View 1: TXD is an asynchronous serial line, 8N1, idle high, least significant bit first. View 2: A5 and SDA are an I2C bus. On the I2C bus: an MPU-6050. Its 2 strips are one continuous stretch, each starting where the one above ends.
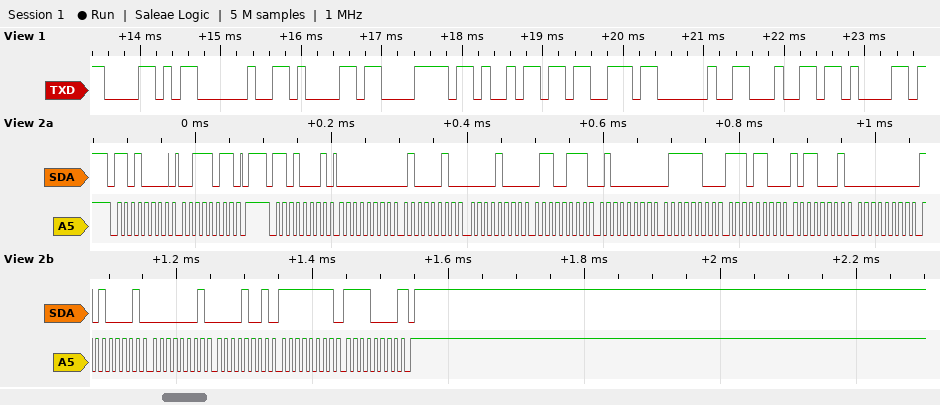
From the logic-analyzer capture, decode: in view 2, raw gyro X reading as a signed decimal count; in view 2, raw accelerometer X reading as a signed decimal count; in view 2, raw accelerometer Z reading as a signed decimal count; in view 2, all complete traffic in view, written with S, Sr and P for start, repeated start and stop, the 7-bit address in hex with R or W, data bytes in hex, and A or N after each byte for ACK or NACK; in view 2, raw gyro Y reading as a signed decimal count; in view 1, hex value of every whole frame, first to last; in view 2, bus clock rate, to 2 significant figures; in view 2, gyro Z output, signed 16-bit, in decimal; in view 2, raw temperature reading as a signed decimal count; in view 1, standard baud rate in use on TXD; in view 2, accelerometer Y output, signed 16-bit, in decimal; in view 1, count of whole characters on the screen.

161
66
16508
S 68W A 3B A P S 68R A 00 A 42 A 08 A 67 A 40 A 7C A EC A B1 A 00 A A1 A 01 A 09 A FF A F0 N P
265
58 20 61 78 69 73 20 64 61
100 kHz
-16
-4943
9600 baud
2151
9
